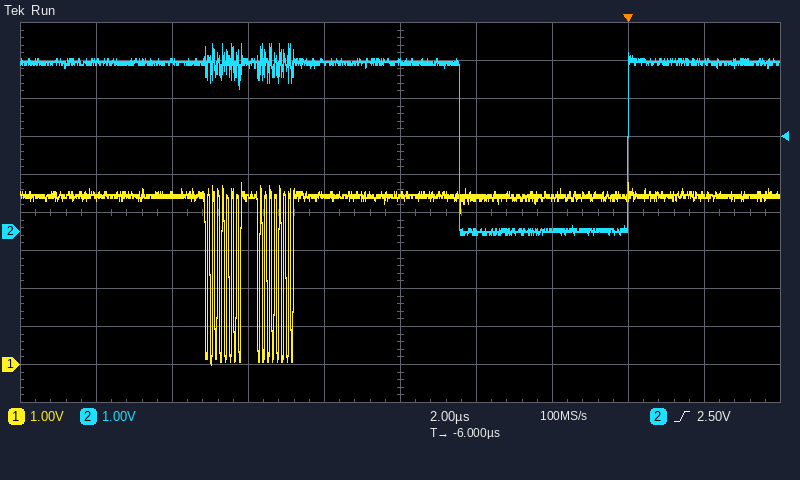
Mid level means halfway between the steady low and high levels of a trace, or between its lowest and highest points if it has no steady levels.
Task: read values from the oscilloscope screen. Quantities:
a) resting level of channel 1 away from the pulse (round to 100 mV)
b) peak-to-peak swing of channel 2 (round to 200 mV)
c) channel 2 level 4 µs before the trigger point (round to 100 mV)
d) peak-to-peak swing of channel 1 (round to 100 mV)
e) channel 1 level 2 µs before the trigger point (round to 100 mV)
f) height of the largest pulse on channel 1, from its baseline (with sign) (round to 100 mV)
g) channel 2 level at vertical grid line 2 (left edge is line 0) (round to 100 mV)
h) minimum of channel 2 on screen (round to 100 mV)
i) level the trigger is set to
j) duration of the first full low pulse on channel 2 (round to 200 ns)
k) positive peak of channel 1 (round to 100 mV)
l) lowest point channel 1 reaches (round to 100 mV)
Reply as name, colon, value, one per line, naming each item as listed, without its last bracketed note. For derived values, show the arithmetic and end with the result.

resting level of channel 1 away from the pulse: 4.4 V
peak-to-peak swing of channel 2: 5.0 V
channel 2 level 4 µs before the trigger point: 0.0 V
peak-to-peak swing of channel 1: 4.8 V − (0.0 V) = 4.8 V
channel 1 level 2 µs before the trigger point: 4.4 V
height of the largest pulse on channel 1, from its baseline (with sign): 0.0 V − (4.4 V) = -4.4 V
channel 2 level at vertical grid line 2 (left edge is line 0): 4.5 V
minimum of channel 2 on screen: -100 mV
level the trigger is set to: 2.50 V
duration of the first full low pulse on channel 2: 4.4 µs
positive peak of channel 1: 4.8 V
lowest point channel 1 reaches: 0.0 V
